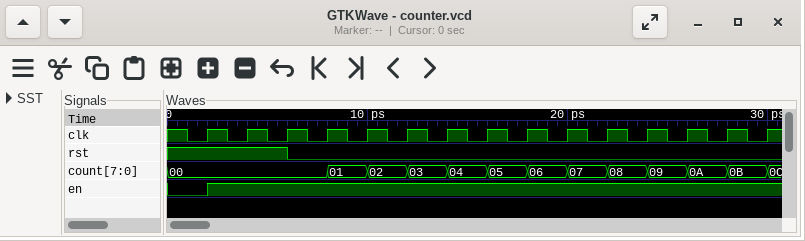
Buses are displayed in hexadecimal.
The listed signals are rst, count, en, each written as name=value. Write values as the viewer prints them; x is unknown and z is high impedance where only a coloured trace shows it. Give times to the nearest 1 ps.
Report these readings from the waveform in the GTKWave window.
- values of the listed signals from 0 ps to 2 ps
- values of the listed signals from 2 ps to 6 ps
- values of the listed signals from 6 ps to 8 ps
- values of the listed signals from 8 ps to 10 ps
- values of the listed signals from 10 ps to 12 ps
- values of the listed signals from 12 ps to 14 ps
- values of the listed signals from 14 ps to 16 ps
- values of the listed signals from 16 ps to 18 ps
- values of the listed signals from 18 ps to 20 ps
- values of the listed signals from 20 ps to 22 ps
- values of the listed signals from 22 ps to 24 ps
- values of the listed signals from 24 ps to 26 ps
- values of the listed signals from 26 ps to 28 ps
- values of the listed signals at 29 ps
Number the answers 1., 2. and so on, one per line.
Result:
1. rst=1, count=00, en=0
2. rst=1, count=00, en=1
3. rst=0, count=00, en=1
4. rst=0, count=01, en=1
5. rst=0, count=02, en=1
6. rst=0, count=03, en=1
7. rst=0, count=04, en=1
8. rst=0, count=05, en=1
9. rst=0, count=06, en=1
10. rst=0, count=07, en=1
11. rst=0, count=08, en=1
12. rst=0, count=09, en=1
13. rst=0, count=0A, en=1
14. rst=0, count=0B, en=1
